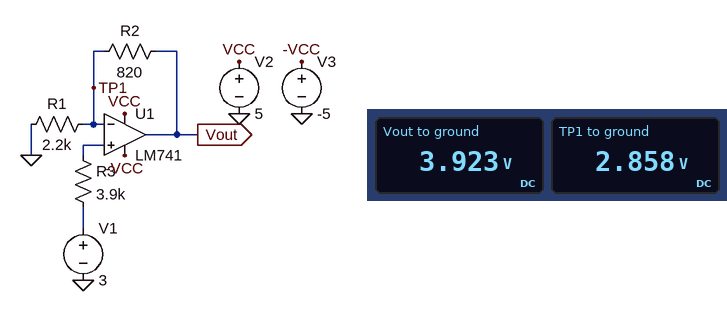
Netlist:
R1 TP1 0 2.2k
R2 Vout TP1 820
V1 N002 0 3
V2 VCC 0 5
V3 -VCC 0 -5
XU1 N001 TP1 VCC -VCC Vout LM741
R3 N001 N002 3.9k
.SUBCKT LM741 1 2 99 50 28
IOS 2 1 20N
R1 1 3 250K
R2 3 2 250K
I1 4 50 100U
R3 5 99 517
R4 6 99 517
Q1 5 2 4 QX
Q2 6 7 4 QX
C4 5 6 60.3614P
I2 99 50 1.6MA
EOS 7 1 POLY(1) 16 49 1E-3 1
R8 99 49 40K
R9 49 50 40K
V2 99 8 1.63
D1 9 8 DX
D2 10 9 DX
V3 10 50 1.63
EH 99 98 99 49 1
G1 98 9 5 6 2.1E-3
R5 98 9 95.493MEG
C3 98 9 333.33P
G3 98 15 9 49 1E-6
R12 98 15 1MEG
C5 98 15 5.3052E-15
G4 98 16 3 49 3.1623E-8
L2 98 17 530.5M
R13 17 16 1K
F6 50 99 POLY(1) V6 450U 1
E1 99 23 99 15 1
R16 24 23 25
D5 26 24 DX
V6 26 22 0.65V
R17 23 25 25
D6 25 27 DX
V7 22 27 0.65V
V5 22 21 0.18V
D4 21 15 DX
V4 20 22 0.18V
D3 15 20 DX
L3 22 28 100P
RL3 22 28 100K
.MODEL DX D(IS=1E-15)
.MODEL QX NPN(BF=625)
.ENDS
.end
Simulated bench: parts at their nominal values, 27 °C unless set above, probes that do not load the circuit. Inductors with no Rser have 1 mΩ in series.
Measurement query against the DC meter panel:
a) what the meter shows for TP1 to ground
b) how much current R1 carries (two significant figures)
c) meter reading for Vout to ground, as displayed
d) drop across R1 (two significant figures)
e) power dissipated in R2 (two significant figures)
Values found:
2.858 V
1.3 mA
3.923 V
2.9 V
1.4 mW
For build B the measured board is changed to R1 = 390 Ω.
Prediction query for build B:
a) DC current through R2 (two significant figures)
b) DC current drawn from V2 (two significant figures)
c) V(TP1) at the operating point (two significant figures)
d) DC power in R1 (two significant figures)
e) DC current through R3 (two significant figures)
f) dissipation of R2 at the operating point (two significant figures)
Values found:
3.2 mA
4.6 mA
1.2 V
4.0 mW
3.6 µA
8.3 mW
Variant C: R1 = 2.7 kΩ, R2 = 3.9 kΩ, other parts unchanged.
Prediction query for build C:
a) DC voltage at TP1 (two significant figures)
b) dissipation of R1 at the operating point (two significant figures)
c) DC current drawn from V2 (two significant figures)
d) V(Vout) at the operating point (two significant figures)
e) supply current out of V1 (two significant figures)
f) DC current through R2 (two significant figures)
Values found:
1.6 V
980 µW
2.0 mA
4.0 V
2.9 µA
600 µA
